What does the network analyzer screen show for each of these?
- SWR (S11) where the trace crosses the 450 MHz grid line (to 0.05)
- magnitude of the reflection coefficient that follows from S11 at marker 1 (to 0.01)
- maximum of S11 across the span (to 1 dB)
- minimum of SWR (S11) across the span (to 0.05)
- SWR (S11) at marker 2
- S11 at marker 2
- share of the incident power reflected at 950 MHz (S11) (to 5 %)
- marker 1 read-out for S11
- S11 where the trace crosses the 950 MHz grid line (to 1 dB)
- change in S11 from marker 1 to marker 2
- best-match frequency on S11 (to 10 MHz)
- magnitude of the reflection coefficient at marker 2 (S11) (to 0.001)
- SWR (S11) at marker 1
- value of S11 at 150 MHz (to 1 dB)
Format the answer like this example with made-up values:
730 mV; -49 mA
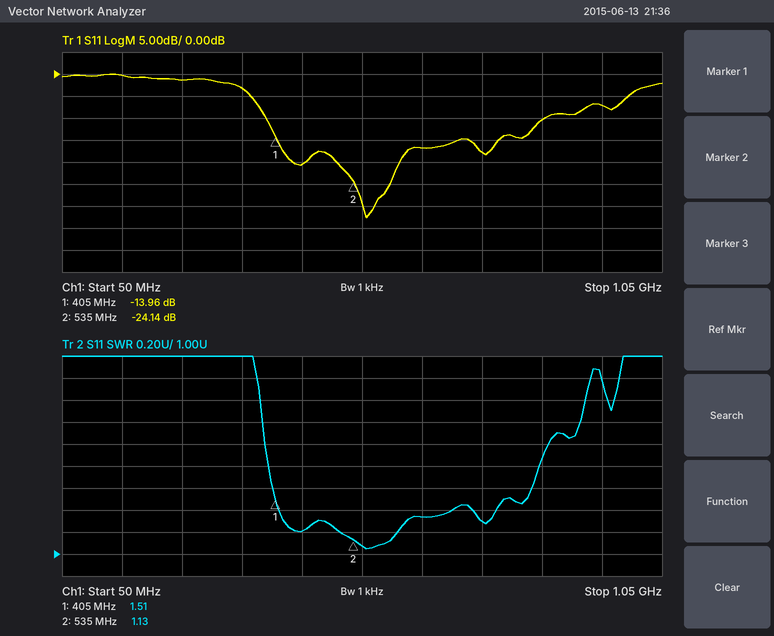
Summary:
1.20; 0.20; 0 dB; 1.05; 1.13; -24.14 dB; 20 %; -13.96 dB; -7 dB; -10.18 dB; 560 MHz; 0.062; 1.51; 0 dB
